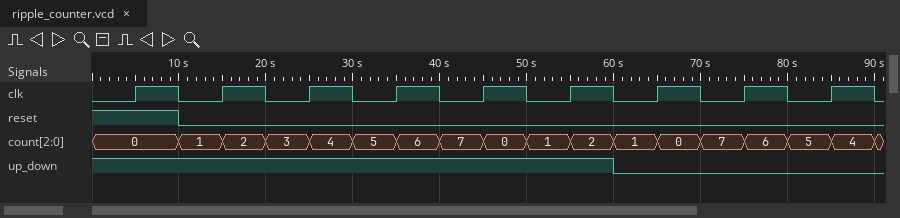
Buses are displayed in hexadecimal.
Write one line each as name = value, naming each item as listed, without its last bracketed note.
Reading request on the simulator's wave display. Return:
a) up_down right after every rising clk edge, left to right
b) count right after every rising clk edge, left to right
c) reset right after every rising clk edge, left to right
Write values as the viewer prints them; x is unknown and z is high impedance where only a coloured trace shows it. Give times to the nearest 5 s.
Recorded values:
up_down right after every rising clk edge, left to right = 1 1 1 1 1 1 0 0 0
count right after every rising clk edge, left to right = 0, 2, 4, 6, 0, 2, 0, 6, 4
reset right after every rising clk edge, left to right = 1 0 0 0 0 0 0 0 0
